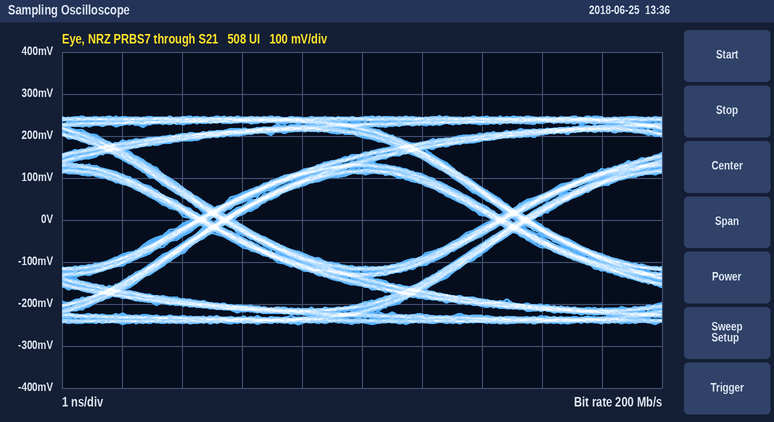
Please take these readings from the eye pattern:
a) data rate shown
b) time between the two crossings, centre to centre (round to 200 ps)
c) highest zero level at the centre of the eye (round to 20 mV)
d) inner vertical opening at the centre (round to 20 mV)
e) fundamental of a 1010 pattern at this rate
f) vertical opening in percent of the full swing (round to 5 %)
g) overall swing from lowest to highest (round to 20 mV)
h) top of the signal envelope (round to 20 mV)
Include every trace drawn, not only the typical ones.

200 Mb/s
5.0 ns
-120 mV
220 mV
100 MHz
45 %
500 mV
240 mV
